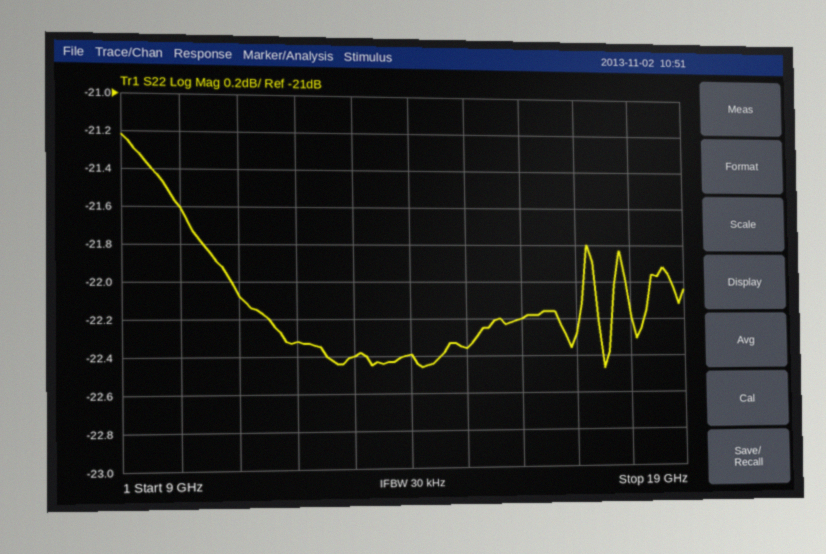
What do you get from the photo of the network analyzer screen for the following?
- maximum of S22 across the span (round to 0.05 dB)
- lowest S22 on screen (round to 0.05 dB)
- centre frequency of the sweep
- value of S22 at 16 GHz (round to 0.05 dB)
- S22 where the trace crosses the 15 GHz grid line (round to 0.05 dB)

-21.20 dB
-22.45 dB
14 GHz
-22.20 dB
-22.35 dB
